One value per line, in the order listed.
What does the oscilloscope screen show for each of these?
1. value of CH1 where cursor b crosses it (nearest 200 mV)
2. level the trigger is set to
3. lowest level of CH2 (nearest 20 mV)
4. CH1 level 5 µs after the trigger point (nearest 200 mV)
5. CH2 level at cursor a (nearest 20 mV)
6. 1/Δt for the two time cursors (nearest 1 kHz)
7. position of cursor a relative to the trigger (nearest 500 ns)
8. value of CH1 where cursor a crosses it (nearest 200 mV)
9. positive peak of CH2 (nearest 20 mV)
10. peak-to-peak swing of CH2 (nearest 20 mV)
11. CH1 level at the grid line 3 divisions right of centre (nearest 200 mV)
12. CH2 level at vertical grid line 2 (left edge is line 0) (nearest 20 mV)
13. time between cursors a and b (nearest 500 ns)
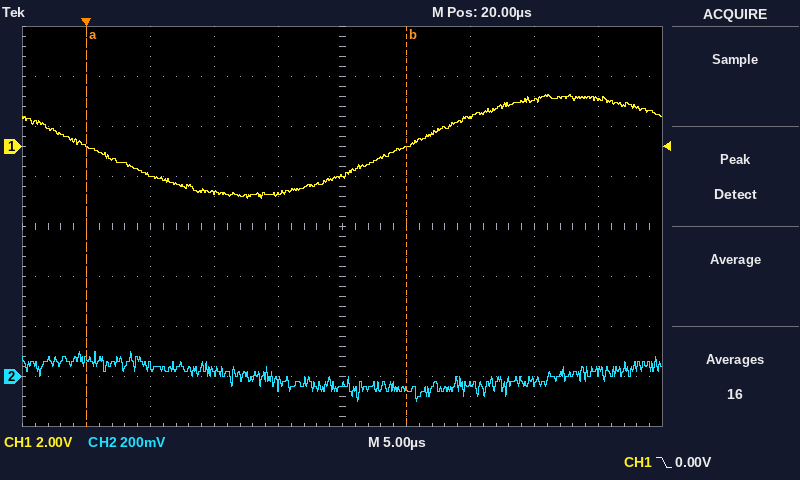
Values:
0.0 V
0.00 V
-100 mV
-1.2 V
60 mV
40 kHz
0.0 µs
0.0 V
100 mV
200 mV
1.8 V
40 mV
25.0 µs
